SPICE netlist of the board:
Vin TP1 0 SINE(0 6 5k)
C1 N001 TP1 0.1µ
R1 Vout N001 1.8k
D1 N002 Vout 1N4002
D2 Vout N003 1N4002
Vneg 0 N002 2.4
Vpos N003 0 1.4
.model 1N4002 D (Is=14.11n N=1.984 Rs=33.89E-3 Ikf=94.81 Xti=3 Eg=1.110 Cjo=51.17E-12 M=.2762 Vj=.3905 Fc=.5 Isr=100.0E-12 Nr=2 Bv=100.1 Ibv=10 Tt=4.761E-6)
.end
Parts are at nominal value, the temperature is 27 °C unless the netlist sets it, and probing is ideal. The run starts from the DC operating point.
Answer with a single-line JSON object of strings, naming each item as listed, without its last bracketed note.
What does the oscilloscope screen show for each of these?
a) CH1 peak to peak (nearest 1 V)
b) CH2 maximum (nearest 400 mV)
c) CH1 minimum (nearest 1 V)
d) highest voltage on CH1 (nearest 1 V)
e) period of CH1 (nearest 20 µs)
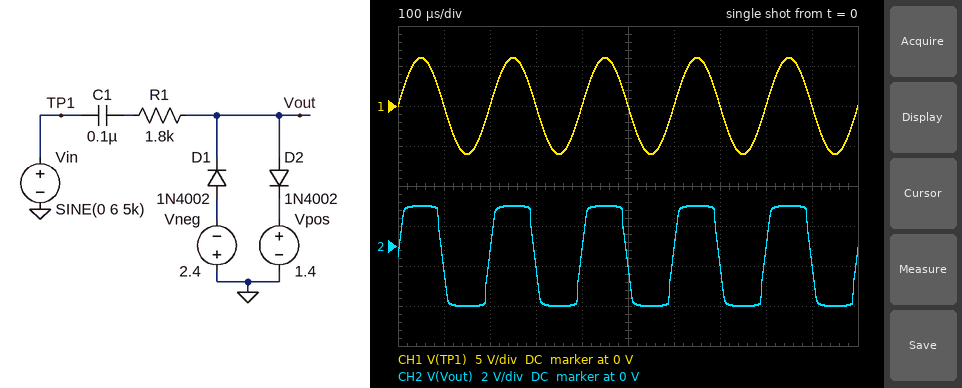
{"CH1 peak to peak": "12 V", "CH2 maximum": "2.0 V", "CH1 minimum": "-6 V", "highest voltage on CH1": "6 V", "period of CH1": "200 µs"}
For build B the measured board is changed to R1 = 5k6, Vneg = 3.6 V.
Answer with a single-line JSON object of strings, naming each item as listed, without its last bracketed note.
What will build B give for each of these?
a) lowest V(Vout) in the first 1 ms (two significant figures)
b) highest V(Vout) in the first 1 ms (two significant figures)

{"lowest V(Vout) in the first 1 ms": "-4.1 V", "highest V(Vout) in the first 1 ms": "1.9 V"}
